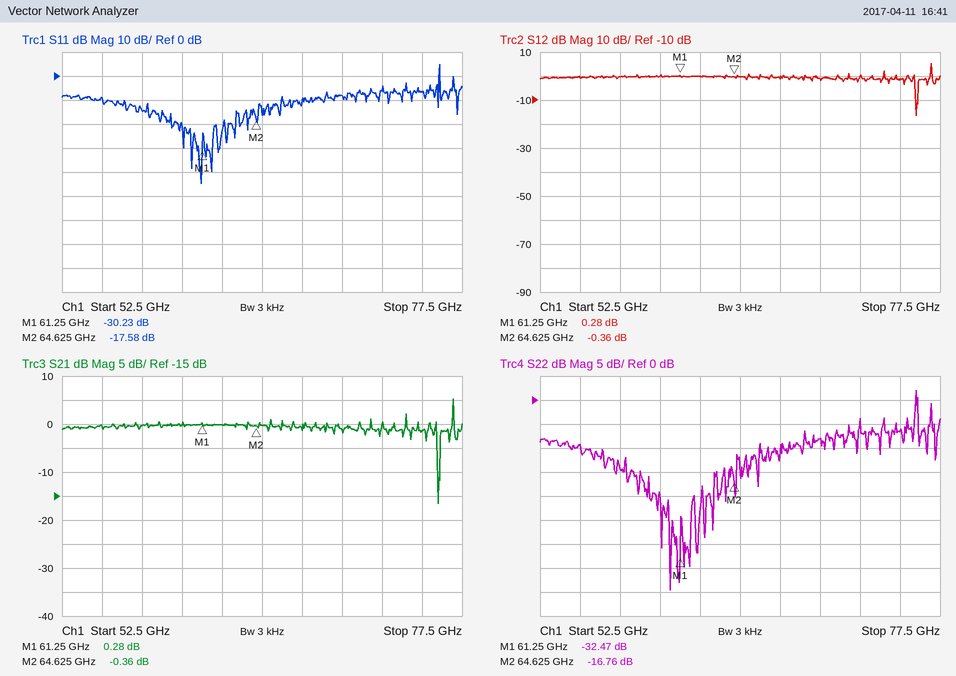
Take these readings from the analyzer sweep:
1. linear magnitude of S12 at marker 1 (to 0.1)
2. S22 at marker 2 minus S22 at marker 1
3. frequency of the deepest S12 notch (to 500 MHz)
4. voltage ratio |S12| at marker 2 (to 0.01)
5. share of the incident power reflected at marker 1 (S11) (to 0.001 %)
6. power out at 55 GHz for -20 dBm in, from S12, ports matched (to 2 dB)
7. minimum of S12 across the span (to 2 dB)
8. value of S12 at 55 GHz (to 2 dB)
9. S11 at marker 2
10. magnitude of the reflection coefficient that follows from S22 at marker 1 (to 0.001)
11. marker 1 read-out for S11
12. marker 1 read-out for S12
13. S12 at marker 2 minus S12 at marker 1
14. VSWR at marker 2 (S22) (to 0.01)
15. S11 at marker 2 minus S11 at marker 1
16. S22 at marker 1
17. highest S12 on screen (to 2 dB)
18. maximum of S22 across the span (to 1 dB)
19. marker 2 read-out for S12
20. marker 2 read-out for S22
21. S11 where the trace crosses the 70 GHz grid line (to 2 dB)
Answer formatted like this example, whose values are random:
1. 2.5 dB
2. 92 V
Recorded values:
1. 1.0
2. 15.71 dB
3. 76.0 GHz
4. 0.96
5. 0.095 %
6. -20 dBm
7. -16 dB
8. 0 dB
9. -17.58 dB
10. 0.024
11. -30.23 dB
12. 0.28 dB
13. -0.64 dB
14. 1.34
15. 12.65 dB
16. -32.47 dB
17. 6 dB
18. 2 dB
19. -0.36 dB
20. -16.76 dB
21. -8 dB
